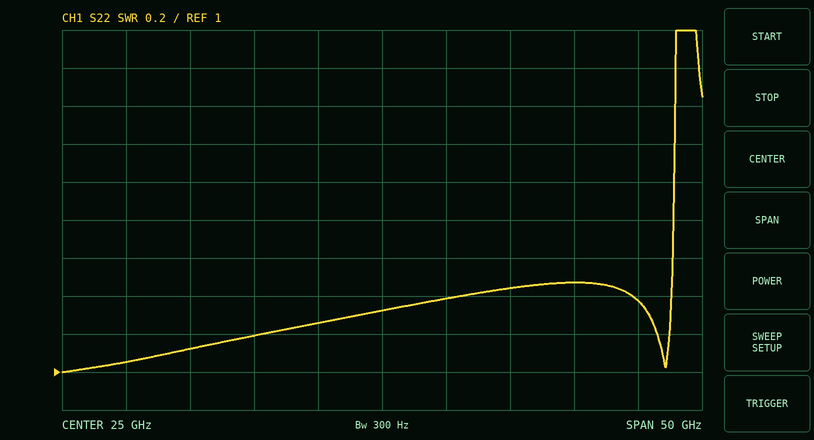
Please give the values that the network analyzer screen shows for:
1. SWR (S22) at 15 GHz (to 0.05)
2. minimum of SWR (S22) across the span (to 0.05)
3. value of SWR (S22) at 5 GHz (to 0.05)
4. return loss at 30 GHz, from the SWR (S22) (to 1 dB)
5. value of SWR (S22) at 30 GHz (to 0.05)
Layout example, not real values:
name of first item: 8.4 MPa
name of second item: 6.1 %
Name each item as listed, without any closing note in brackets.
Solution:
SWR (S22) at 15 GHz: 1.20
minimum of SWR (S22) across the span: 1.00
value of SWR (S22) at 5 GHz: 1.05
return loss at 30 GHz, from the SWR (S22): 16 dB
value of SWR (S22) at 30 GHz: 1.40
